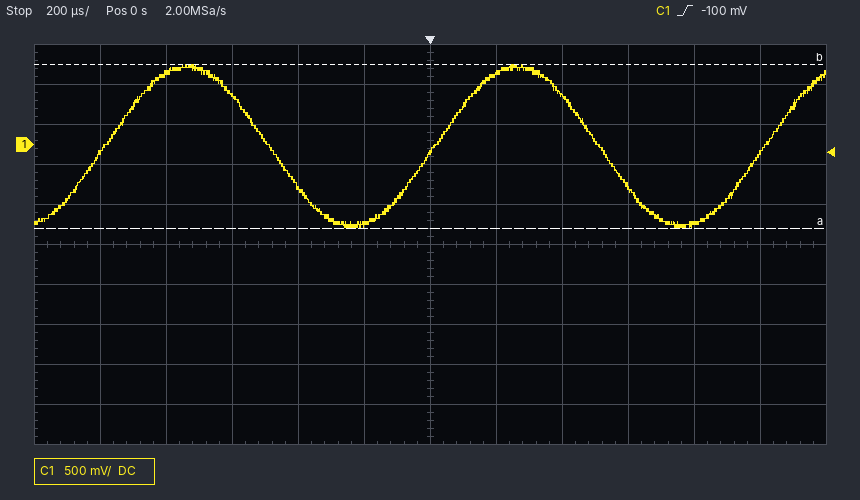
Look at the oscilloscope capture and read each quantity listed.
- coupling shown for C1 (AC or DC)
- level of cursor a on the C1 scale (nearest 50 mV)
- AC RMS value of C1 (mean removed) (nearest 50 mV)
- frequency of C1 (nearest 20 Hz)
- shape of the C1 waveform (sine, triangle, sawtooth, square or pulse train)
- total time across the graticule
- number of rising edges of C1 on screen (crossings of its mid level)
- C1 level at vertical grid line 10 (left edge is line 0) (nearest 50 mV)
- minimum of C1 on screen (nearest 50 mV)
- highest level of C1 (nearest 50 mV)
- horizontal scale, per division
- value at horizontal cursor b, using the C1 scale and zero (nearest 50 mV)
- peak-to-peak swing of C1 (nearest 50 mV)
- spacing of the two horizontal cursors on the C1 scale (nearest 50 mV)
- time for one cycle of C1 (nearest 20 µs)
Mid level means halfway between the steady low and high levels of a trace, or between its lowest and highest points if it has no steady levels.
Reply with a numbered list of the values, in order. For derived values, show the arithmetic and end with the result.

1. DC
2. -1.05 V
3. 2.05 V / (2√2) ≈ 725 mV, so 700 mV to the nearest 50 mV
4. 1 / 1.00 ms ≈ 1.00 kHz
5. sine
6. 2.4 ms
7. 3
8. -1.00 V
9. -1.05 V
10. 1.00 V
11. 200 µs
12. 1.00 V
13. 1.00 V − (-1.05 V) = 2.05 V
14. 2.05 V
15. 1.00 ms
